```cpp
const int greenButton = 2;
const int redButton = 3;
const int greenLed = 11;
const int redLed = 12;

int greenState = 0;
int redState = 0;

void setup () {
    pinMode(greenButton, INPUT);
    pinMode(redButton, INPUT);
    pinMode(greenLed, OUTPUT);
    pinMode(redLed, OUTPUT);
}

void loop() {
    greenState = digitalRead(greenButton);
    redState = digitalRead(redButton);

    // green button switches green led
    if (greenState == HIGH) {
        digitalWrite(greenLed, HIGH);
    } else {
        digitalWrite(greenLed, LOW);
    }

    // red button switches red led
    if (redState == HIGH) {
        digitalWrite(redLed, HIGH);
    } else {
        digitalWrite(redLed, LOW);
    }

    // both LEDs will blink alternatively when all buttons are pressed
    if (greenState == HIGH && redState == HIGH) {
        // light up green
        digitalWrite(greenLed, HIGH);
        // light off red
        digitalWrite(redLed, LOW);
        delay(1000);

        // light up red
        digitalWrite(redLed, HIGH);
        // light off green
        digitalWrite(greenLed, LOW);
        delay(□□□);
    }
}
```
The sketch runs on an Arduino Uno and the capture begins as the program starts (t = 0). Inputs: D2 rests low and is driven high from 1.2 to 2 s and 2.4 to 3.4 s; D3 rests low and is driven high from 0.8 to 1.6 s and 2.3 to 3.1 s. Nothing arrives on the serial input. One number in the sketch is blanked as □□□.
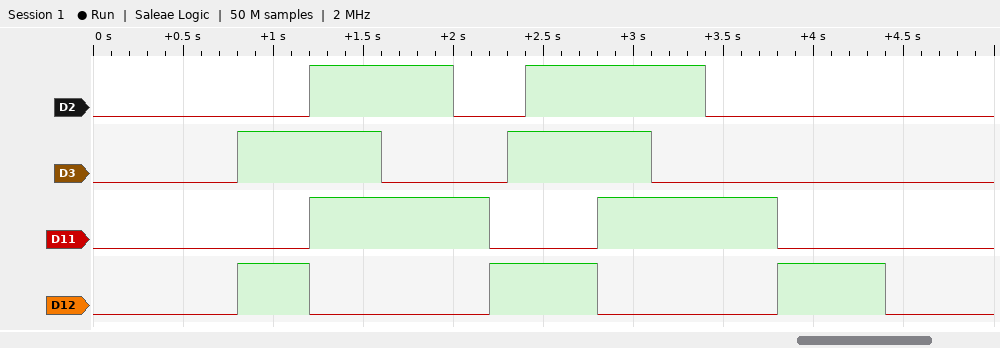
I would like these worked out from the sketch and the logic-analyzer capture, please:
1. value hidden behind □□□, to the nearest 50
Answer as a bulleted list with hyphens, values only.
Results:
- 600
